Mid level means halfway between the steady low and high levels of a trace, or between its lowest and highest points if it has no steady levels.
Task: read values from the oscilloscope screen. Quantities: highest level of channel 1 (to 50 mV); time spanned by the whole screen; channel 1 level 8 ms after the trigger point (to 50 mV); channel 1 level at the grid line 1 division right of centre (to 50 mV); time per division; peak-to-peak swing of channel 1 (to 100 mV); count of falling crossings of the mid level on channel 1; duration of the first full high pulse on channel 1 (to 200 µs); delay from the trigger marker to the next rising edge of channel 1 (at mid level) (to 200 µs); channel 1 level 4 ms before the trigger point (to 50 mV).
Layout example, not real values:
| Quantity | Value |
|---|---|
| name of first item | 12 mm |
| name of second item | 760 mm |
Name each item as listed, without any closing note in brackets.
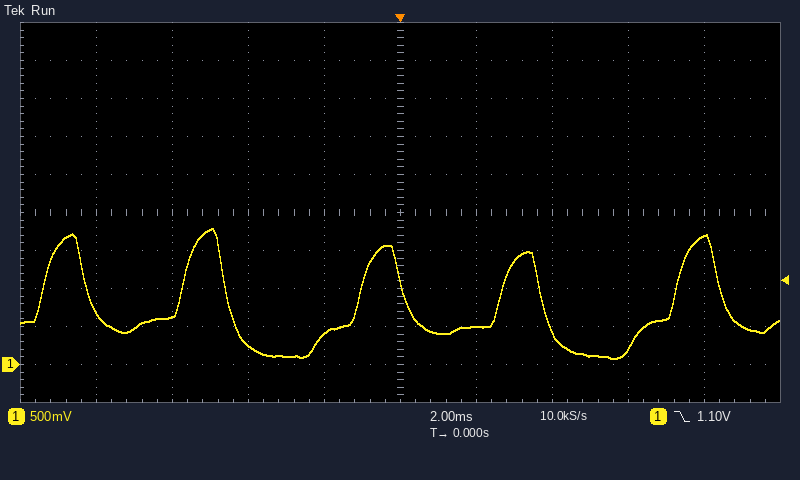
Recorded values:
| Quantity | Value |
|---|---|
| highest level of channel 1 | 1.80 V |
| time spanned by the whole screen | 20 ms |
| channel 1 level 8 ms after the trigger point | 1.70 V |
| channel 1 level at the grid line 1 division right of centre | 500 mV |
| time per division | 2 ms |
| peak-to-peak swing of channel 1 | 1.70 V |
| count of falling crossings of the mid level on channel 1 | 5 |
| duration of the first full high pulse on channel 1 | 1.2 ms |
| delay from the trigger marker to the next rising edge of channel 1 (at mid level) | 2.6 ms |
| channel 1 level 4 ms before the trigger point | 250 mV |
